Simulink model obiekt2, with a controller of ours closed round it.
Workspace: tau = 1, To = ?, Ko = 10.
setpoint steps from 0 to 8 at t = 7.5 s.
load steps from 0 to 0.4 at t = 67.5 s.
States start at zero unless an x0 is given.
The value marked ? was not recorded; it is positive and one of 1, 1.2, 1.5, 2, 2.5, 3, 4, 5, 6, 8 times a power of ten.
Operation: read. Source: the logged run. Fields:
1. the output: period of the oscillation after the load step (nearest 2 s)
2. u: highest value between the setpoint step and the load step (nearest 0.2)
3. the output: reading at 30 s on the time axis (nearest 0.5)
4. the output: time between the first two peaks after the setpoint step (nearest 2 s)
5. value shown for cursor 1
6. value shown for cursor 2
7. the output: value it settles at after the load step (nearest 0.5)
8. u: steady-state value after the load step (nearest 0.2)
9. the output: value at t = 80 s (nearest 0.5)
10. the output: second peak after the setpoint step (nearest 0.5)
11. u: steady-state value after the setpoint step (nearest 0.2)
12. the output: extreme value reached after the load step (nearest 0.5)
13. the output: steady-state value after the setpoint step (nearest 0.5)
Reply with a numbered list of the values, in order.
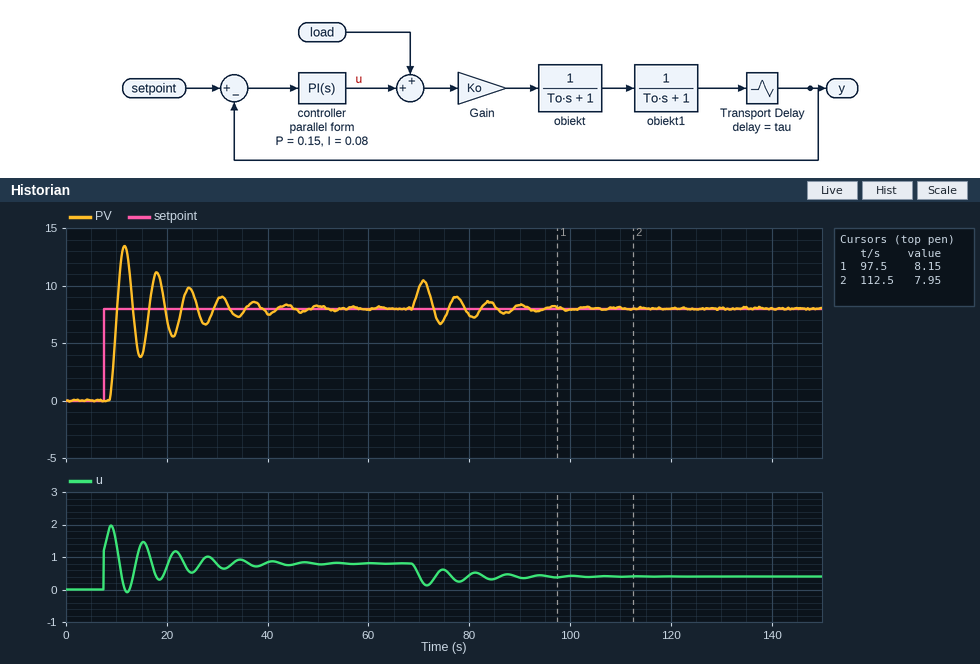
1. 6 s
2. 2.0
3. 8.5
4. 6 s
5. 8.15
6. 7.95
7. 8.0
8. 0.4
9. 7.5
10. 11.0
11. 0.8
12. 10.5
13. 8.0
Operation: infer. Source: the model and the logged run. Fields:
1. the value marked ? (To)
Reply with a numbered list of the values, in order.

1. 1
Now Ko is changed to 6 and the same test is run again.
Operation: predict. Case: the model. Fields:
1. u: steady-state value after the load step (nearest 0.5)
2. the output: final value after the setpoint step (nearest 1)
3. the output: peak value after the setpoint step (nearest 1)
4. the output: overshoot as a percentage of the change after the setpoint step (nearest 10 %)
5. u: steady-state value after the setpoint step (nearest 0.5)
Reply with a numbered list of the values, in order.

1. 1.0
2. 8
3. 10
4. 20 %
5. 1.5
